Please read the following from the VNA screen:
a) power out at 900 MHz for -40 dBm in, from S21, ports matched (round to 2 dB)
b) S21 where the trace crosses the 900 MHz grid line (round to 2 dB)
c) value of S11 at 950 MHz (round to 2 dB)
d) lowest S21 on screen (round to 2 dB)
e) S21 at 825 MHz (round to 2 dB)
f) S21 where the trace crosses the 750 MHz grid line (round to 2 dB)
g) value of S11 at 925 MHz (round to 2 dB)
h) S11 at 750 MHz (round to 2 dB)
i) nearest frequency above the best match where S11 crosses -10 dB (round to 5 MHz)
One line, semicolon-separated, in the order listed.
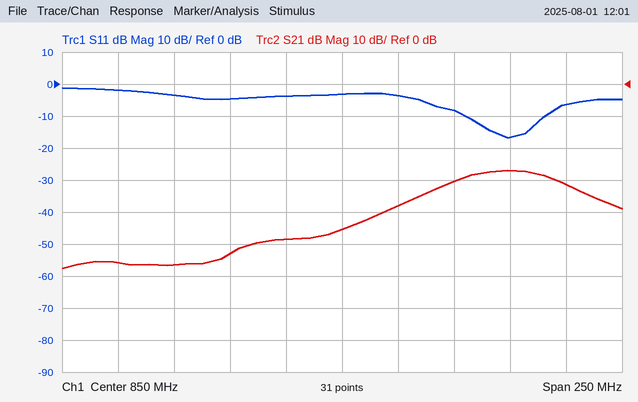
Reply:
-70 dBm; -30 dB; -6 dB; -58 dB; -48 dB; -56 dB; -16 dB; -2 dB; 940 MHz
